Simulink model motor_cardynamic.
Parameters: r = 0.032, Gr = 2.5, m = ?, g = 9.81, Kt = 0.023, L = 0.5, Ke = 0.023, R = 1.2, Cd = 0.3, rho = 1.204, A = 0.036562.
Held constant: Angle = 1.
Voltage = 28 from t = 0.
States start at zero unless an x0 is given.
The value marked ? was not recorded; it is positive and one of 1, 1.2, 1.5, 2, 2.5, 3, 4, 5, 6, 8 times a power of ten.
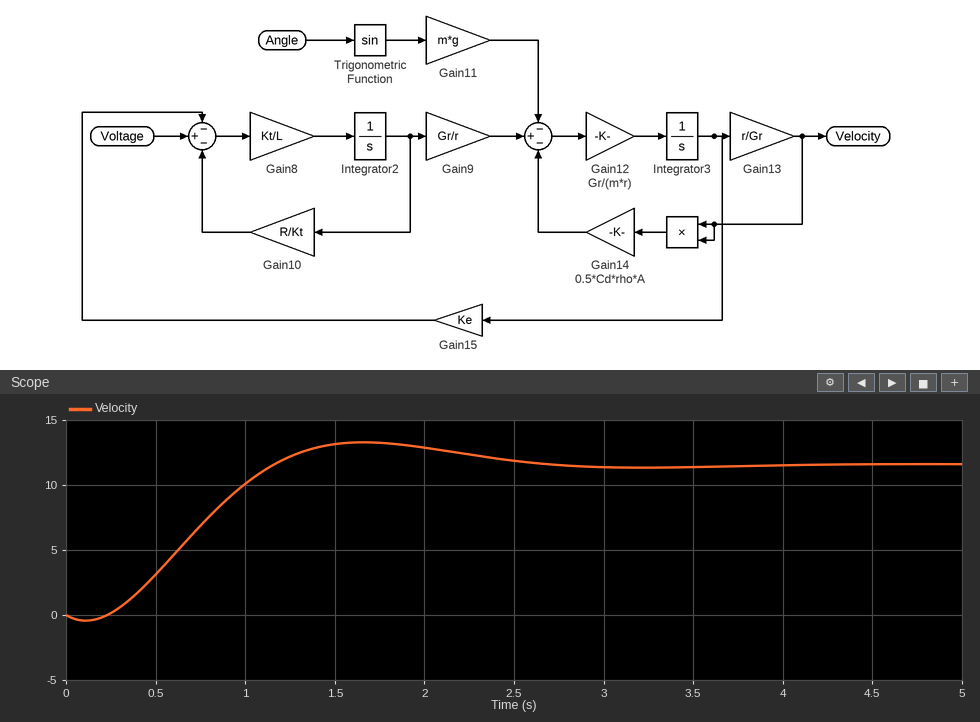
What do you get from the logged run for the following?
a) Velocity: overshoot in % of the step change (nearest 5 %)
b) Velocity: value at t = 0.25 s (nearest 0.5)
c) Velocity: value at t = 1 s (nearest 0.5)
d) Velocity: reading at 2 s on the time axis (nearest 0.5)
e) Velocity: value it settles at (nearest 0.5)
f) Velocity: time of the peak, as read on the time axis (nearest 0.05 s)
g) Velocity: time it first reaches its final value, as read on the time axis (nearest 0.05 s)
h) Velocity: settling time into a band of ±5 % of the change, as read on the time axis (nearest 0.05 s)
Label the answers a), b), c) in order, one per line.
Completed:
a) 15 %
b) 0.0
c) 10.0
d) 13.0
e) 11.5
f) 1.65 s
g) 1.15 s
h) 2.35 s
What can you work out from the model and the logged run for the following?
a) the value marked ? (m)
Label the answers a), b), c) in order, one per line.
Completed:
a) 1.2
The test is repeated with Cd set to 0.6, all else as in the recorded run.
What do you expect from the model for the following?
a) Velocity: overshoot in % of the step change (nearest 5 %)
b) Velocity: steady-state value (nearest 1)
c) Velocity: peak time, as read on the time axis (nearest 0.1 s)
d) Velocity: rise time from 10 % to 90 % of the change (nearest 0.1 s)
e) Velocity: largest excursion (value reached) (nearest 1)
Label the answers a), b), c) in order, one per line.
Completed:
a) 15 %
b) 11
c) 1.6 s
d) 0.7 s
e) 13
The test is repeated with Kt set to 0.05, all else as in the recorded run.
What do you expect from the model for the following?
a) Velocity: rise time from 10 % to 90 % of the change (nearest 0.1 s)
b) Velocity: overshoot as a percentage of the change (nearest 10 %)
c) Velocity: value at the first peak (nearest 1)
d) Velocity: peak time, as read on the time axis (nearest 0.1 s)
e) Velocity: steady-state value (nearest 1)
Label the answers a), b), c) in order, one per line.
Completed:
a) 0.4 s
b) 30 %
c) 18
d) 1.0 s
e) 14
